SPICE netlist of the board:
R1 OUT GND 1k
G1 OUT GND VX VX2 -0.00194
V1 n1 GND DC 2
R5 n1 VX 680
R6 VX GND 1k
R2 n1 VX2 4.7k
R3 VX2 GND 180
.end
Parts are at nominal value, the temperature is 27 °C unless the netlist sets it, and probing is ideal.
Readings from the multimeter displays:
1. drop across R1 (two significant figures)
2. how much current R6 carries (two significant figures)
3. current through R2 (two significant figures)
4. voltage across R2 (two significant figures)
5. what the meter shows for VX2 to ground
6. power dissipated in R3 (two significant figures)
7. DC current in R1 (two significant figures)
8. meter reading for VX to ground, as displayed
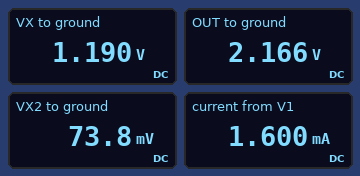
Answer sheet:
2.2 V
1.2 mA
410 µA
1.9 V
73.8 mV
30 µW
2.2 mA
1.190 V
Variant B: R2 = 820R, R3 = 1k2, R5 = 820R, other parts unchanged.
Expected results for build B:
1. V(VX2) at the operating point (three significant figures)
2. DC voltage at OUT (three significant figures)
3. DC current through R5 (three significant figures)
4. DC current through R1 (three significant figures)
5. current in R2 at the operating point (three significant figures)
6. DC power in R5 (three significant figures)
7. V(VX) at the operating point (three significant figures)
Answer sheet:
1.19 V
-173 mV
1.10 mA
173 µA
990 µA
990 µW
1.10 V
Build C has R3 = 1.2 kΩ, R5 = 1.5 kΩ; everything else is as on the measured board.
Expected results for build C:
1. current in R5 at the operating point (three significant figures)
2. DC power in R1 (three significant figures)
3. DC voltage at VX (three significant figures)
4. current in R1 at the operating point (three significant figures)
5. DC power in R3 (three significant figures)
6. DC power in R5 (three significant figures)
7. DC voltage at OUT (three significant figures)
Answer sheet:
800 µA
582 µW
800 mV
763 µA
138 µW
960 µW
763 mV
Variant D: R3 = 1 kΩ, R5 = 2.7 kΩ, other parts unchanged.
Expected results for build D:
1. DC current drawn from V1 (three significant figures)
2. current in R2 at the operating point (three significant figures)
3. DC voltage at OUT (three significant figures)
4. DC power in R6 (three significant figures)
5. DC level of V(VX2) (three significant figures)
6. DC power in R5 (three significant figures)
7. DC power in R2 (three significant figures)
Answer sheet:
891 µA
351 µA
368 mV
292 µW
351 mV
789 µW
579 µW
